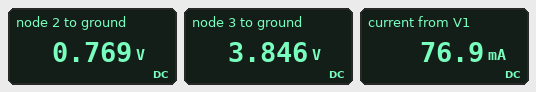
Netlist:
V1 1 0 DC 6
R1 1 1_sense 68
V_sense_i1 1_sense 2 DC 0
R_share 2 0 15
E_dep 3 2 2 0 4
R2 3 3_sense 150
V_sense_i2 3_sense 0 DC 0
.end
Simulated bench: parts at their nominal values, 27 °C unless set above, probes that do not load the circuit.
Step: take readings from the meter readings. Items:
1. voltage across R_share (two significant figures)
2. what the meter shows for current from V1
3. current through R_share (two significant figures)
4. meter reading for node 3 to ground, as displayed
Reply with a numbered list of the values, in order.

1. 770 mV
2. 76.9 mA
3. 51 mA
4. 3.846 V
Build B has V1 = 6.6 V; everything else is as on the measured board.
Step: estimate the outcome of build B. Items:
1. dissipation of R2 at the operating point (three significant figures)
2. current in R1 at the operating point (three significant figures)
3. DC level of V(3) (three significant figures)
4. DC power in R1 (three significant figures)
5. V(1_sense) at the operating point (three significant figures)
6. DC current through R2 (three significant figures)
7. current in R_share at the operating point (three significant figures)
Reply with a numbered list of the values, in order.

1. 119 mW
2. 84.6 mA
3. 4.23 V
4. 487 mW
5. 846 mV
6. 28.2 mA
7. 56.4 mA
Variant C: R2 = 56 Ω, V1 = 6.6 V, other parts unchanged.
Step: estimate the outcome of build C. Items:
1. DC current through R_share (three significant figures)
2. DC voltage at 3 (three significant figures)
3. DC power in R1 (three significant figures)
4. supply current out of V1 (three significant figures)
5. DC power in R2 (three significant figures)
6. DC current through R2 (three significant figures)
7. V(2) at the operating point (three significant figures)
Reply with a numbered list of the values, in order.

1. 37.9 mA
2. 2.84 V
3. 535 mW
4. 88.7 mA
5. 144 mW
6. 50.8 mA
7. 569 mV
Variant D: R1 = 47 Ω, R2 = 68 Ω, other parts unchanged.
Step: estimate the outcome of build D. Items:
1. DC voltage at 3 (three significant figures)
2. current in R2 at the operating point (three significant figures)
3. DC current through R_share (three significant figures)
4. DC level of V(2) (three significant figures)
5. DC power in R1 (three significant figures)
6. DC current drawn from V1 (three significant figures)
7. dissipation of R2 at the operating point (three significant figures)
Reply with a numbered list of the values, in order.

1. 3.95 V
2. 58.1 mA
3. 52.7 mA
4. 791 mV
5. 577 mW
6. 111 mA
7. 230 mW
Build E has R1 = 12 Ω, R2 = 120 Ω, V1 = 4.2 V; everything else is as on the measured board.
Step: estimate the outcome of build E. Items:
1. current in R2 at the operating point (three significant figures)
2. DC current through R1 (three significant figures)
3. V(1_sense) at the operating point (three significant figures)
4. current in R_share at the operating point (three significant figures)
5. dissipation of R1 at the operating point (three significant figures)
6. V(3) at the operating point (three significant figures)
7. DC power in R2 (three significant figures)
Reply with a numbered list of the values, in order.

1. 76.1 mA
2. 198 mA
3. 1.83 V
4. 122 mA
5. 470 mW
6. 9.13 V
7. 695 mW
